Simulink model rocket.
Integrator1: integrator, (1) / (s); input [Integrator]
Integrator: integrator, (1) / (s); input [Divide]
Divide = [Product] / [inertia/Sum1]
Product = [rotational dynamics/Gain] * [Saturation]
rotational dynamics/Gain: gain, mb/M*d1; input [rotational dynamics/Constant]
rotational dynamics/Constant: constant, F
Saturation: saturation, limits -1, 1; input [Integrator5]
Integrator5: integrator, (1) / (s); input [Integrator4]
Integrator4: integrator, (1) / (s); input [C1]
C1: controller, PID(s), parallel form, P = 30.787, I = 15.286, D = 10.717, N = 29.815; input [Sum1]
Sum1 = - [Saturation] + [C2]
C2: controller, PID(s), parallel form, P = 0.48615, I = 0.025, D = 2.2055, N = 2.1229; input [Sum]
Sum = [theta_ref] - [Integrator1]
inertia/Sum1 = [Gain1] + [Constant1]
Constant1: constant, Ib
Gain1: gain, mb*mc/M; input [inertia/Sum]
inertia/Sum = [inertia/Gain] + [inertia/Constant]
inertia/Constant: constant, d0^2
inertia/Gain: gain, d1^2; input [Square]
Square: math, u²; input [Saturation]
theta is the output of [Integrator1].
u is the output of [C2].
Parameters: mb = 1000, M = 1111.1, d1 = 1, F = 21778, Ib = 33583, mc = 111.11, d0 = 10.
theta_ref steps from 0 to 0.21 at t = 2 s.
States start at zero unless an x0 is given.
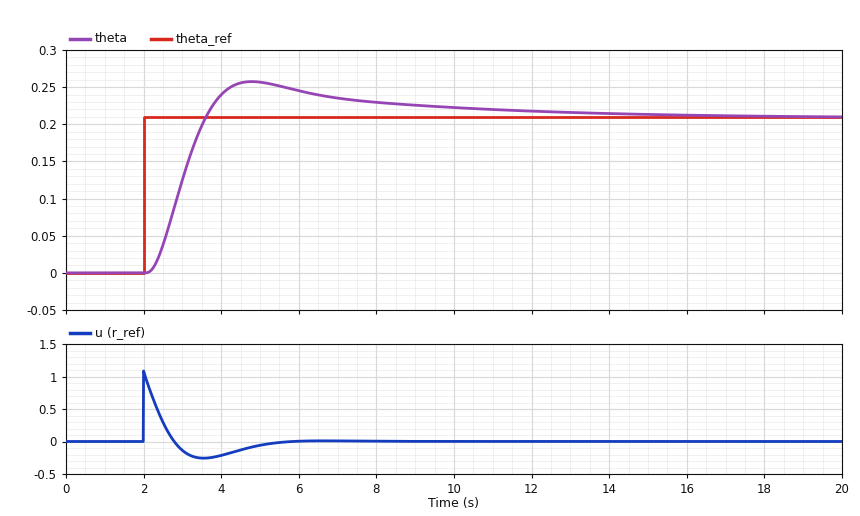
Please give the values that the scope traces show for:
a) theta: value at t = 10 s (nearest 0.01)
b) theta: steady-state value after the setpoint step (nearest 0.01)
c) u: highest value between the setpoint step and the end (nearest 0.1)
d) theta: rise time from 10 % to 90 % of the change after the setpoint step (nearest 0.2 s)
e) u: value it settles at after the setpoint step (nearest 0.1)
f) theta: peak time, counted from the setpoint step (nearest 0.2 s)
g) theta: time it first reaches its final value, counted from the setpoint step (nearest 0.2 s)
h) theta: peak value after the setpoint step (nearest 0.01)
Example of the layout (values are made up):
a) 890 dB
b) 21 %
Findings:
a) 0.22
b) 0.21
c) 1.1
d) 1.0 s
e) 0.0
f) 2.8 s
g) 1.6 s
h) 0.26
